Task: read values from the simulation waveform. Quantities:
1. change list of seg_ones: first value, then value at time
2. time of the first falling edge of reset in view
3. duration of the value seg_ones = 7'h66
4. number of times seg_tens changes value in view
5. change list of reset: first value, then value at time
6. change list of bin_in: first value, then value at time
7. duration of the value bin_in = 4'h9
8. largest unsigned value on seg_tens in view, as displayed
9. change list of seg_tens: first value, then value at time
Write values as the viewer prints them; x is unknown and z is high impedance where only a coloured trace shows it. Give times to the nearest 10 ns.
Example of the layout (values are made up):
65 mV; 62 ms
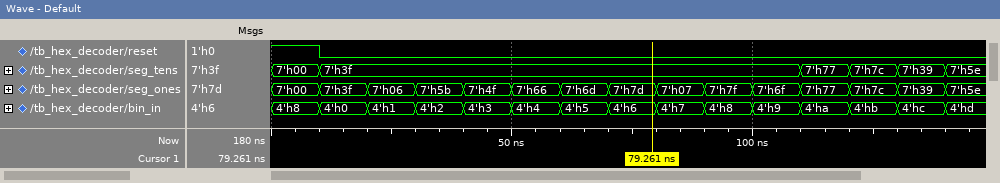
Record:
7'h00, 7'h3f at 10 ns, 7'h06 at 20 ns, 7'h5b at 30 ns, 7'h4f at 40 ns, 7'h66 at 50 ns, 7'h6d at 60 ns, 7'h7d at 70 ns, 7'h07 at 80 ns, 7'h7f at 90 ns, 7'h6f at 100 ns, 7'h77 at 110 ns, 7'h7c at 120 ns, 7'h39 at 130 ns, 7'h5e at 140 ns; 10 ns; 10 ns; 5; 1, 0 at 10 ns; 4'h8, 4'h0 at 10 ns, 4'h1 at 20 ns, 4'h2 at 30 ns, 4'h3 at 40 ns, 4'h4 at 50 ns, 4'h5 at 60 ns, 4'h6 at 70 ns, 4'h7 at 80 ns, 4'h8 at 90 ns, 4'h9 at 100 ns, 4'ha at 110 ns, 4'hb at 120 ns, 4'hc at 130 ns, 4'hd at 140 ns; 10 ns; 7'h7c; 7'h00, 7'h3f at 10 ns, 7'h77 at 110 ns, 7'h7c at 120 ns, 7'h39 at 130 ns, 7'h5e at 140 ns
